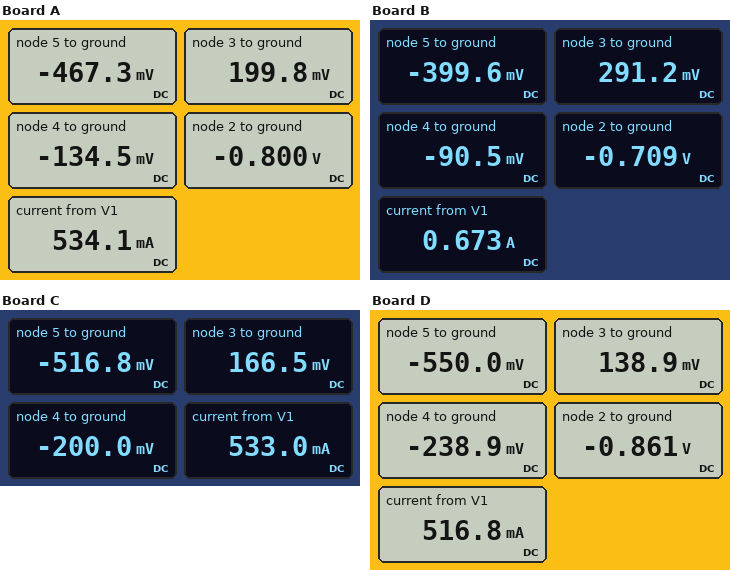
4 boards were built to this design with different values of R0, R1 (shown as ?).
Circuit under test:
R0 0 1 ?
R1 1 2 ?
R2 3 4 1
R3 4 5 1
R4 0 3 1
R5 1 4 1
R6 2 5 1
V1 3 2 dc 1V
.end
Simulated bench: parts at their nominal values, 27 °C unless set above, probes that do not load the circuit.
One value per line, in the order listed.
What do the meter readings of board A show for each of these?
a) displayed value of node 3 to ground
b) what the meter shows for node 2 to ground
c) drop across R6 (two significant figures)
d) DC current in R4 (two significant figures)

199.8 mV
-0.800 V
330 mV
200 mA
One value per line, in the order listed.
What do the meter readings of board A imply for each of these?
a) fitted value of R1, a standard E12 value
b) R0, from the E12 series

3.3 Ω
0.68 Ω
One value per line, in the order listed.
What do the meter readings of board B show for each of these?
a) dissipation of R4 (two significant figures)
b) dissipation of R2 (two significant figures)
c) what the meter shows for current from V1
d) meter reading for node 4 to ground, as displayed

85 mW
150 mW
0.673 A
-90.5 mV
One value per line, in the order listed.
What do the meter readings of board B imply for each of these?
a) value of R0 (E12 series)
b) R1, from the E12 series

0.56 Ω
1.5 Ω
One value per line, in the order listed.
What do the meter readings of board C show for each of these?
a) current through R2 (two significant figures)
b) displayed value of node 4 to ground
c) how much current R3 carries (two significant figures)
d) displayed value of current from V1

370 mA
-200.0 mV
320 mA
533.0 mA
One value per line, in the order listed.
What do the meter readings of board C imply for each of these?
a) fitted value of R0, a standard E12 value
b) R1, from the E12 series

1.5 Ω
2.7 Ω
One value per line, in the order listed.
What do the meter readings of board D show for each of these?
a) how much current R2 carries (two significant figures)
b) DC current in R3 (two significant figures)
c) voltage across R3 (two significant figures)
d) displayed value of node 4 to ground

380 mA
310 mA
310 mV
-238.9 mV
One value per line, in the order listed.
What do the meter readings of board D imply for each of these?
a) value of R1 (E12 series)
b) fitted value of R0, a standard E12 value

2.7 Ω
2.2 Ω
